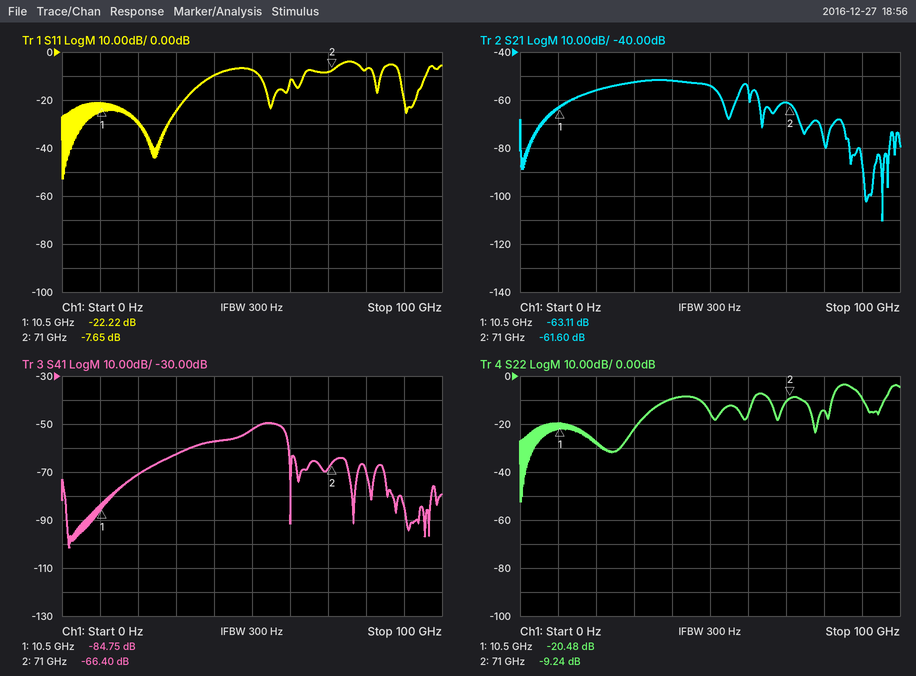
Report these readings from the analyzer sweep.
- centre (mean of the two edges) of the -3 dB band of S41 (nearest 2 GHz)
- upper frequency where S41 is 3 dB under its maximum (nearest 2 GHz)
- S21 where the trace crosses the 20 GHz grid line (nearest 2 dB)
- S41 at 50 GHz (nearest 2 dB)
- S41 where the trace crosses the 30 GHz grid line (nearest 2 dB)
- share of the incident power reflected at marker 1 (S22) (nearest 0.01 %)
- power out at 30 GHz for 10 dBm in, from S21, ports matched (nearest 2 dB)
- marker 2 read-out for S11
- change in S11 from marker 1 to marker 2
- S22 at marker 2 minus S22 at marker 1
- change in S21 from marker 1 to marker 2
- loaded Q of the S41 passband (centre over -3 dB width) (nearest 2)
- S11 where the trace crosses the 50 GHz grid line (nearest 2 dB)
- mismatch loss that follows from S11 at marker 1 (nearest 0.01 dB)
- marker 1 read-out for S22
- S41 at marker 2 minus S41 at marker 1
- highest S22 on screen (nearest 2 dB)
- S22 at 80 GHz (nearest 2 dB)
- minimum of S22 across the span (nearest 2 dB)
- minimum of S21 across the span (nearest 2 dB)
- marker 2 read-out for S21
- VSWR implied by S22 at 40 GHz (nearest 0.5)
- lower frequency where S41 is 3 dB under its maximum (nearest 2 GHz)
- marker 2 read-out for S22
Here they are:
54 GHz
58 GHz
-56 dB
-52 dB
-62 dB
0.90 %
-42 dBm
-7.65 dB
14.57 dB
11.24 dB
1.51 dB
6
-8 dB
0.03 dB
-20.48 dB
18.35 dB
-4 dB
-14 dB
-52 dB
-110 dB
-61.60 dB
2.0
50 GHz
-9.24 dB
